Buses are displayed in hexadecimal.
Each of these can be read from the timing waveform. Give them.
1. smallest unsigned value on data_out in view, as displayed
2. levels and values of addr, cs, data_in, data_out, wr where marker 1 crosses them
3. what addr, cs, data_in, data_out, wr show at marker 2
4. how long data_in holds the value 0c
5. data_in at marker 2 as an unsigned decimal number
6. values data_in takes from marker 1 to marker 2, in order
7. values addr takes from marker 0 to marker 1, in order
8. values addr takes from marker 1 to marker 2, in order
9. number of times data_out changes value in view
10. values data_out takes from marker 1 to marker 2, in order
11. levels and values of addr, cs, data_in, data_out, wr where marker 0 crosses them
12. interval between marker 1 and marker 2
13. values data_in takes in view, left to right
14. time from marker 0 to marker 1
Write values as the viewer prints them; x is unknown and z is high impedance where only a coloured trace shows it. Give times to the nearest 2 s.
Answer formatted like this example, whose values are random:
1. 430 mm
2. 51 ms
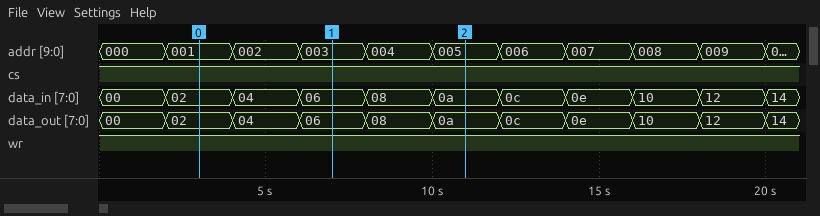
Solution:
1. 00
2. addr=003, cs=1, data_in=06, data_out=06, wr=1
3. addr=005, cs=1, data_in=0a, data_out=0a, wr=1
4. 2 s
5. 10
6. 06, 08, 0a
7. 001, 002, 003
8. 003, 004, 005
9. 10
10. 06, 08, 0a
11. addr=001, cs=1, data_in=02, data_out=02, wr=1
12. 4 s
13. 00, 02, 04, 06, 08, 0a, 0c, 0e, 10, 12, 14
14. 4 s
